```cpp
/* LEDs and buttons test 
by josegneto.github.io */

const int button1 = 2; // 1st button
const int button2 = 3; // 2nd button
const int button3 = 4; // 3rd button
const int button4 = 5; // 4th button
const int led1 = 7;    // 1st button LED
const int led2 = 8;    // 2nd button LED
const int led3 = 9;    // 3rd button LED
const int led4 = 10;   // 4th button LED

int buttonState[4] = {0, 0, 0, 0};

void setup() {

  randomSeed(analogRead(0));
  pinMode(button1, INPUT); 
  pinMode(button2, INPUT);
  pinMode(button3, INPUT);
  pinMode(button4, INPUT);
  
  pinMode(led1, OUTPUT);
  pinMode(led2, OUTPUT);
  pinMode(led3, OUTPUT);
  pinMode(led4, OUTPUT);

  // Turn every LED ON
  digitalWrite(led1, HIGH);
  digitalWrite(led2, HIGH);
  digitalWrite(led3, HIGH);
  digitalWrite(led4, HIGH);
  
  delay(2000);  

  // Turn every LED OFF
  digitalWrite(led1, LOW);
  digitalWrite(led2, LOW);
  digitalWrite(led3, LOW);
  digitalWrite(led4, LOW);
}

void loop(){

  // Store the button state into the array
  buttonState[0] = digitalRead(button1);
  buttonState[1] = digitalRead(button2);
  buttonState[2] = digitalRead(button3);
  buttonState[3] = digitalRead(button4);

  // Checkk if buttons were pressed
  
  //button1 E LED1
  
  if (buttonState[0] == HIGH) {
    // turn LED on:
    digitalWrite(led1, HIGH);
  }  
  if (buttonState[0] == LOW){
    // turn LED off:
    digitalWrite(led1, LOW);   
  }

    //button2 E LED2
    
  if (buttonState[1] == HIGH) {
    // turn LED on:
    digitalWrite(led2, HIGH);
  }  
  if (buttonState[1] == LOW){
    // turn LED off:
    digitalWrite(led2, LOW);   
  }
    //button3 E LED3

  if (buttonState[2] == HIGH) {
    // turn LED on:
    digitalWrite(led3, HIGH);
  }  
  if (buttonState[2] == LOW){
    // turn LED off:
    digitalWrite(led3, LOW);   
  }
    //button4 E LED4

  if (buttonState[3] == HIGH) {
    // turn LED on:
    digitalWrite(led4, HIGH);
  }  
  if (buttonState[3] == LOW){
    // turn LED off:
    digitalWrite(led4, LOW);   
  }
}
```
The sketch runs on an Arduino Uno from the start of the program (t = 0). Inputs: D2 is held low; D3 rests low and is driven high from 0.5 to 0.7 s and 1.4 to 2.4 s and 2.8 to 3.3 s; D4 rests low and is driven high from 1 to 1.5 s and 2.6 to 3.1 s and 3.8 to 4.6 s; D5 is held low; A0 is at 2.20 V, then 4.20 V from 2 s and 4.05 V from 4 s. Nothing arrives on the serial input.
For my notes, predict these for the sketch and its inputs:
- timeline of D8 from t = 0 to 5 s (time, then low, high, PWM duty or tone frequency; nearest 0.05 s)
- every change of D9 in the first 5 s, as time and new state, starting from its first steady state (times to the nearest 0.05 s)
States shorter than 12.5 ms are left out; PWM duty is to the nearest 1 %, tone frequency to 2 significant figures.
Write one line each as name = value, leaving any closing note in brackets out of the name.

timeline of D8 from t = 0 to 5 s = 0 s high; 2.4 s low; 2.8 s high; 3.3 s low
every change of D9 in the first 5 s, as time and new state, starting from its first steady state = 0 s high; 2 s low; 2.6 s high; 3.1 s low; 3.8 s high; 4.6 s low
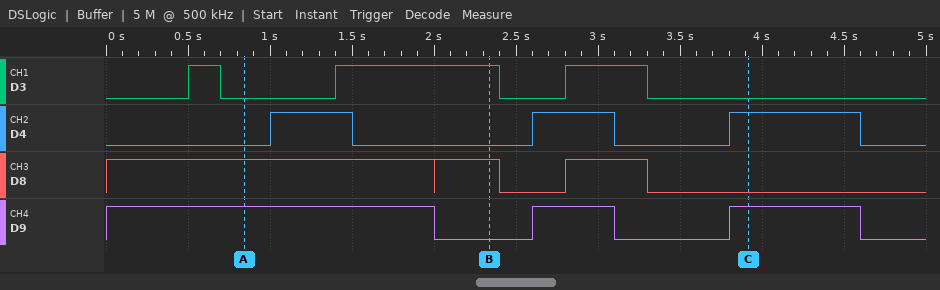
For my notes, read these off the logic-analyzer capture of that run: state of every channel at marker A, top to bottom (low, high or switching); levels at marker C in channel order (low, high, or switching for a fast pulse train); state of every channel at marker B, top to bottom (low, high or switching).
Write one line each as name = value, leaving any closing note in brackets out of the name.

state of every channel at marker A, top to bottom = D3 low, D4 low, D8 high, D9 high
levels at marker C in channel order = D3 low, D4 high, D8 low, D9 high
state of every channel at marker B, top to bottom = D3 high, D4 low, D8 high, D9 low
